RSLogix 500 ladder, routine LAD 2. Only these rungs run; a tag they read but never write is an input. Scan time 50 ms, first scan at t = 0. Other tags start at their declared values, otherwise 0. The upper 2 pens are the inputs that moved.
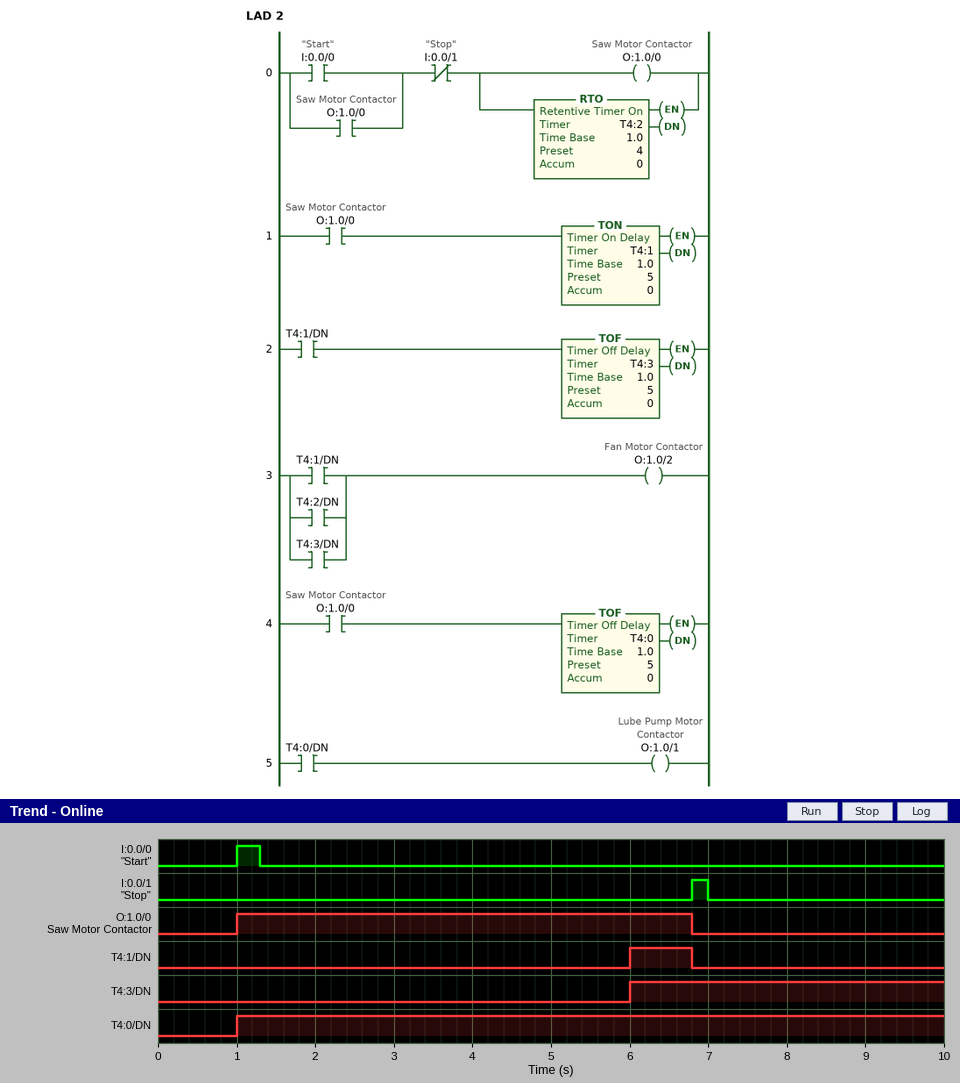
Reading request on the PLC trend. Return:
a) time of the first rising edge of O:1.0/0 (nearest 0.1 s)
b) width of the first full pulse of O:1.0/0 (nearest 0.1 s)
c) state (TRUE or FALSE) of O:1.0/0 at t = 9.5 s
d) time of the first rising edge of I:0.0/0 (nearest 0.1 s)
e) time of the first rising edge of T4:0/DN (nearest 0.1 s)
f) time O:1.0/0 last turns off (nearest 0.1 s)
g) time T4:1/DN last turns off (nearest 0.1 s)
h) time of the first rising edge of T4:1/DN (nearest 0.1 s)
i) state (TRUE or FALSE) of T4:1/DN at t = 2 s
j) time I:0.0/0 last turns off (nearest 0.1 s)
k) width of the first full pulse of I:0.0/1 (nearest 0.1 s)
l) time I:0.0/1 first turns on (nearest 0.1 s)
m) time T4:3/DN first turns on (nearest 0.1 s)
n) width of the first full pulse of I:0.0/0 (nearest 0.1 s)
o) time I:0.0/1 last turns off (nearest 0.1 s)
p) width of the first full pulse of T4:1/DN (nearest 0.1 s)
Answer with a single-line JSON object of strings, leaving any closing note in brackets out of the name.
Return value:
{"time of the first rising edge of O:1.0/0": "1.0 s", "width of the first full pulse of O:1.0/0": "5.8 s", "state (TRUE or FALSE) of O:1.0/0 at t = 9.5 s": "FALSE", "time of the first rising edge of I:0.0/0": "1.0 s", "time of the first rising edge of T4:0/DN": "1.0 s", "time O:1.0/0 last turns off": "6.8 s", "time T4:1/DN last turns off": "6.8 s", "time of the first rising edge of T4:1/DN": "6.0 s", "state (TRUE or FALSE) of T4:1/DN at t = 2 s": "FALSE", "time I:0.0/0 last turns off": "1.3 s", "width of the first full pulse of I:0.0/1": "0.2 s", "time I:0.0/1 first turns on": "6.8 s", "time T4:3/DN first turns on": "6.0 s", "width of the first full pulse of I:0.0/0": "0.3 s", "time I:0.0/1 last turns off": "7.0 s", "width of the first full pulse of T4:1/DN": "0.8 s"}
